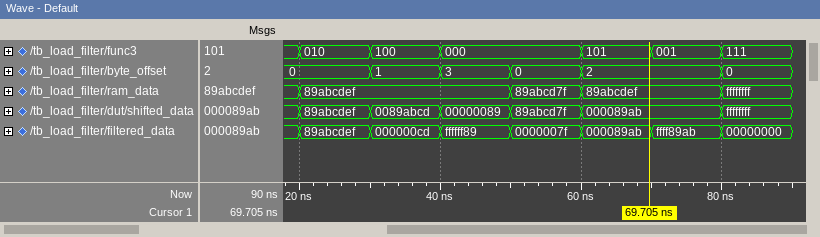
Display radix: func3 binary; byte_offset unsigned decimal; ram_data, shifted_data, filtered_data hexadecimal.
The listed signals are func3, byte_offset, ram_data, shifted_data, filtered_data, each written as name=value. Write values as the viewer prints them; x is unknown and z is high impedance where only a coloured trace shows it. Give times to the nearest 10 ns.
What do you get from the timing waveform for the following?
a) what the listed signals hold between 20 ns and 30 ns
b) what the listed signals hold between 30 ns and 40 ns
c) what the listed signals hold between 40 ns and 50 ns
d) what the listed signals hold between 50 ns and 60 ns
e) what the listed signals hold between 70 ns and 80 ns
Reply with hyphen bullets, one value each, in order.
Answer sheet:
- func3=010, byte_offset=0, ram_data=89abcdef, shifted_data=89abcdef, filtered_data=89abcdef
- func3=100, byte_offset=1, ram_data=89abcdef, shifted_data=0089abcd, filtered_data=000000cd
- func3=000, byte_offset=3, ram_data=89abcdef, shifted_data=00000089, filtered_data=ffffff89
- func3=000, byte_offset=0, ram_data=89abcd7f, shifted_data=89abcd7f, filtered_data=0000007f
- func3=001, byte_offset=2, ram_data=89abcdef, shifted_data=000089ab, filtered_data=ffff89ab
